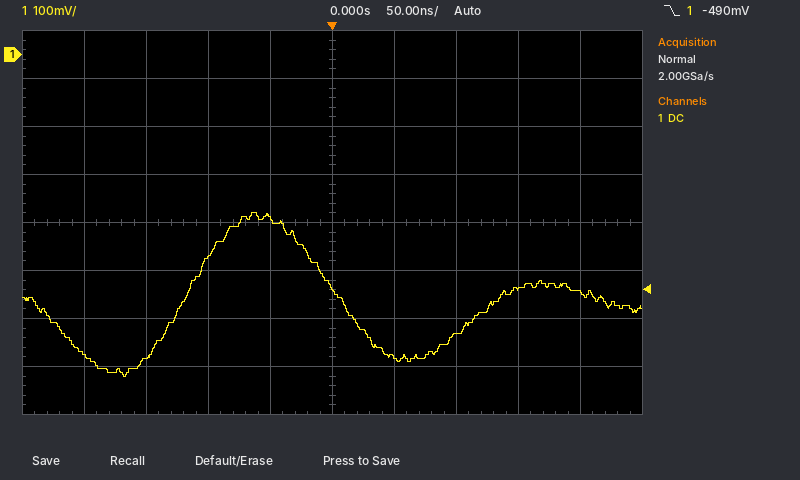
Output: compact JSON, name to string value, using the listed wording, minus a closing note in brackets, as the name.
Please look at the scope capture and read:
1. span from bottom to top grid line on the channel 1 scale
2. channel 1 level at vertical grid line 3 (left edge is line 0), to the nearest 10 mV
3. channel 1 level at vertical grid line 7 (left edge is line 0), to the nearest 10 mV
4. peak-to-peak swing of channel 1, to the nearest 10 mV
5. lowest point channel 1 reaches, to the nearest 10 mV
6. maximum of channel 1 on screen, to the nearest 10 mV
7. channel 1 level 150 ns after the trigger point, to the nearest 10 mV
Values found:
{"span from bottom to top grid line on the channel 1 scale": "800 mV", "channel 1 level at vertical grid line 3 (left edge is line 0), to the nearest 10 mV": "-420 mV", "channel 1 level at vertical grid line 7 (left edge is line 0), to the nearest 10 mV": "-580 mV", "peak-to-peak swing of channel 1, to the nearest 10 mV": "340 mV", "lowest point channel 1 reaches, to the nearest 10 mV": "-670 mV", "maximum of channel 1 on screen, to the nearest 10 mV": "-330 mV", "channel 1 level 150 ns after the trigger point, to the nearest 10 mV": "-490 mV"}
